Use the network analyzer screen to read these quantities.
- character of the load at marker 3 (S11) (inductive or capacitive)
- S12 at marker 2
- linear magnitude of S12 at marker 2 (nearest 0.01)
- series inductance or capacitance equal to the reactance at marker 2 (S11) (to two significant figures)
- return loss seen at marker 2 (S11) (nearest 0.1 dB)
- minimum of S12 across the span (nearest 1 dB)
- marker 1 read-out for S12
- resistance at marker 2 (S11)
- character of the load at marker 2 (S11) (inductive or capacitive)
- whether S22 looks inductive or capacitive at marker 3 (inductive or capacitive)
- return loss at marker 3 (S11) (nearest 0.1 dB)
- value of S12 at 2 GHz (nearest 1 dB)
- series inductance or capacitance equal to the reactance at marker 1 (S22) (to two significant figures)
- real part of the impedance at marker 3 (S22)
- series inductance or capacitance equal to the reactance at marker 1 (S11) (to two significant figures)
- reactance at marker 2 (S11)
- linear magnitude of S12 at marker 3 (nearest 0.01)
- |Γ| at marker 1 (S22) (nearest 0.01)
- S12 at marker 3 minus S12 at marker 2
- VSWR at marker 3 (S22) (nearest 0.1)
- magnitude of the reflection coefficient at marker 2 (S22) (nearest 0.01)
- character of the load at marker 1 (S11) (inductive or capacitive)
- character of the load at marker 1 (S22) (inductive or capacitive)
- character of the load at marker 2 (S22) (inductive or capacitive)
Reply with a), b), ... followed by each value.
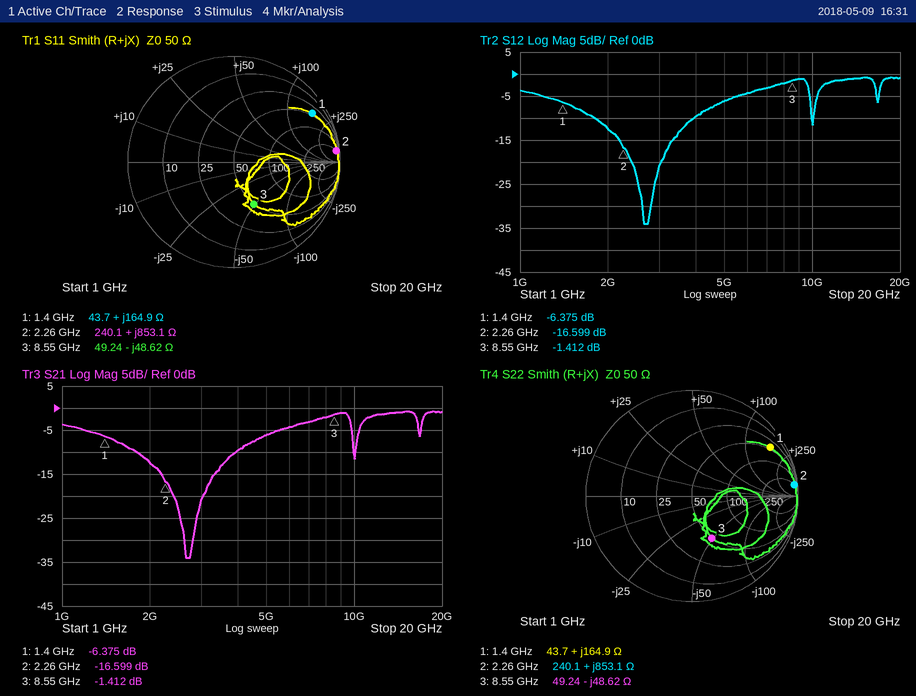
a) capacitive
b) -16.599 dB
c) 0.15
d) 60 nH
e) 0.3 dB
f) -34 dB
g) -6.375 dB
h) 240.1 Ω
i) inductive
j) capacitive
k) 7.1 dB
l) -12 dB
m) 19 nH
n) 49.24 Ω
o) 19 nH
p) +853.1 Ω
q) 0.85
r) 0.87
s) 15.187 dB
t) 2.6
u) 0.97
v) inductive
w) inductive
x) inductive
